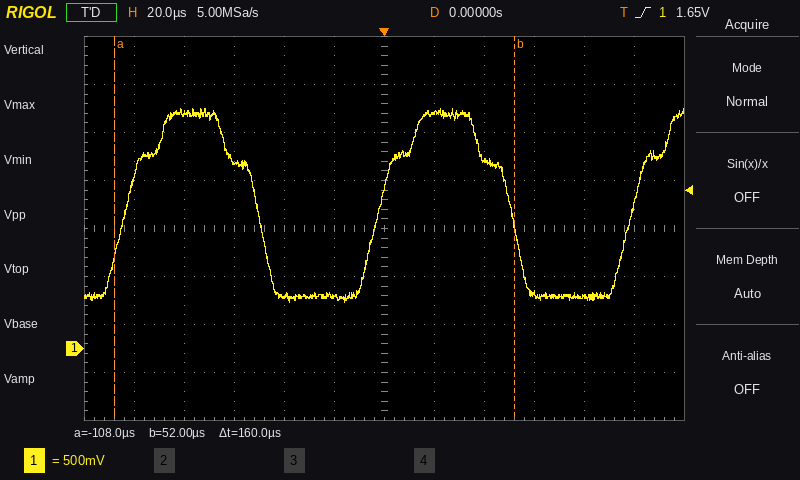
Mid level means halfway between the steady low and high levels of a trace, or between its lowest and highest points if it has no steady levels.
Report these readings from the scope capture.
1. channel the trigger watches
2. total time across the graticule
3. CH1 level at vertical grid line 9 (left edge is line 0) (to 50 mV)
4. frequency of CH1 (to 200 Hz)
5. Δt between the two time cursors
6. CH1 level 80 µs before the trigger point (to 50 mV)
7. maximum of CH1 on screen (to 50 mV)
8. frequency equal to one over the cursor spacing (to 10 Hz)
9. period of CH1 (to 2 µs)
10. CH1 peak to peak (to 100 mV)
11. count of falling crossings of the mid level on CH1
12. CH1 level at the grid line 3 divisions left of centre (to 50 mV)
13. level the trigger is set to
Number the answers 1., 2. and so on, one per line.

1. CH1
2. 240 µs
3. 550 mV
4. 9.8 kHz
5. 160 µs
6. 2.45 V
7. 2.50 V
8. 6.25 kHz
9. 102 µs
10. 2.00 V
11. 2
12. 1.95 V
13. 1.65 V
